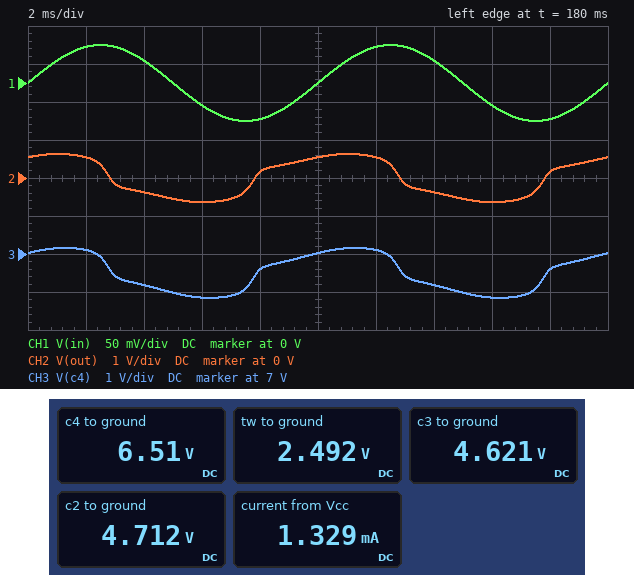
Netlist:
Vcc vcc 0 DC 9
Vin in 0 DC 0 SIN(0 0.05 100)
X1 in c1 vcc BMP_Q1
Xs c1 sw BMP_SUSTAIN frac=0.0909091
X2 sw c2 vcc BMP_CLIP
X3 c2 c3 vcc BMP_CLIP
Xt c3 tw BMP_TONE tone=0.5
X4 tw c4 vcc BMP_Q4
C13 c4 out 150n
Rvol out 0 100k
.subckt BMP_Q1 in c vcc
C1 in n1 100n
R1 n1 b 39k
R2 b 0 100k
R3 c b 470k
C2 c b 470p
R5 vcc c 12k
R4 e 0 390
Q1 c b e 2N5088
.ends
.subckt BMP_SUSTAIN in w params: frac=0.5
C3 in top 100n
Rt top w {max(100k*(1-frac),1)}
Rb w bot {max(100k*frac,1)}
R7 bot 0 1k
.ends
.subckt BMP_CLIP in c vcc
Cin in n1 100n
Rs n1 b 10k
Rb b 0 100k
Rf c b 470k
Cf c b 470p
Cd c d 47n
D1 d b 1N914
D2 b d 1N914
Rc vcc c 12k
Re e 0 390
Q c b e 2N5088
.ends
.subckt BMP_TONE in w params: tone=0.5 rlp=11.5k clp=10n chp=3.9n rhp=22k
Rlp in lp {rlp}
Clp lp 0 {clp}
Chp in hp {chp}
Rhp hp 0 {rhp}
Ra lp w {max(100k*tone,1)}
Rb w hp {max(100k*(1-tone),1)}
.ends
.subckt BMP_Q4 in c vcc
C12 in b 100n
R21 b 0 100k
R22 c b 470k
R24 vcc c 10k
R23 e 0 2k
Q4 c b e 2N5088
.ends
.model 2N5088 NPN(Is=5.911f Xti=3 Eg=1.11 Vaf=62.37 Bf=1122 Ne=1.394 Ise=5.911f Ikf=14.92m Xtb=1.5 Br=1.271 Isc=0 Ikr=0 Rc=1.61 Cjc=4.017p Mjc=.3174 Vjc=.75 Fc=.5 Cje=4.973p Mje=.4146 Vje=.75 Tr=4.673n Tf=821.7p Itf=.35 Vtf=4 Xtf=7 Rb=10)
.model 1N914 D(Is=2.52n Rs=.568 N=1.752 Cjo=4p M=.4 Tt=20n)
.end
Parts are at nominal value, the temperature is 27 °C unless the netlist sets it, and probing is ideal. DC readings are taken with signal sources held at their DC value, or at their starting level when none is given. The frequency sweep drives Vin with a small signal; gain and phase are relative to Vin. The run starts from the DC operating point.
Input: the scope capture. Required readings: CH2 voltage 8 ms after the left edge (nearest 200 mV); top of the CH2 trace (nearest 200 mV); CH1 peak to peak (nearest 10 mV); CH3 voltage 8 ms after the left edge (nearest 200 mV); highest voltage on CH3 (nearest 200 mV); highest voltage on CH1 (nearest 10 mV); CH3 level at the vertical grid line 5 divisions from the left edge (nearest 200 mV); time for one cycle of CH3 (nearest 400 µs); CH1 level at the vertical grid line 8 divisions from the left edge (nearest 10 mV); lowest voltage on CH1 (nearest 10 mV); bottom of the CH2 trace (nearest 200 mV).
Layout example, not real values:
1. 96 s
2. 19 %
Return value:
1. 200 mV
2. 600 mV
3. 100 mV
4. 6.6 V
5. 7.2 V
6. 50 mV
7. 7.0 V
8. 10.0 ms
9. -30 mV
10. -50 mV
11. -600 mV
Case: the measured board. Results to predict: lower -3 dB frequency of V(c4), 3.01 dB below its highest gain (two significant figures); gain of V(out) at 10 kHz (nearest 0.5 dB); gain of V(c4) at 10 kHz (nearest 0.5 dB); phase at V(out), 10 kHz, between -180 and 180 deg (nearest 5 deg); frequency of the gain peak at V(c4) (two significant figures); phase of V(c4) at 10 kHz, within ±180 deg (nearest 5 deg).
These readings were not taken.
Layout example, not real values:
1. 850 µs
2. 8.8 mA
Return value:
1. 71 Hz
2. -8.0 dB
3. -8.0 dB
4. 135 deg
5. 210 Hz
6. 135 deg
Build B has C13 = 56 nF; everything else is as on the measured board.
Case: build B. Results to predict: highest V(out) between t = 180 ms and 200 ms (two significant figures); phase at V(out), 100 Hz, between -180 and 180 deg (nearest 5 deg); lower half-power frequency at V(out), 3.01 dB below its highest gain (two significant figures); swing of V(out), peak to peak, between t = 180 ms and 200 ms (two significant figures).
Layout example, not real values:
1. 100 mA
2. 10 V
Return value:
1. 590 mV
2. 85 deg
3. 76 Hz
4. 1.2 V
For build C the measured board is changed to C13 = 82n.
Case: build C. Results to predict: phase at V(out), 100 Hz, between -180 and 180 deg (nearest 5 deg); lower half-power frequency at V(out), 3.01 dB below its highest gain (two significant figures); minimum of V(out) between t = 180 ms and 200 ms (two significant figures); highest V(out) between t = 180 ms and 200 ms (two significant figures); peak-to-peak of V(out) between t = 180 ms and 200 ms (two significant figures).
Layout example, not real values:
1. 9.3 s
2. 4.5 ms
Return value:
1. 80 deg
2. 74 Hz
3. -620 mV
4. 610 mV
5. 1.2 V
